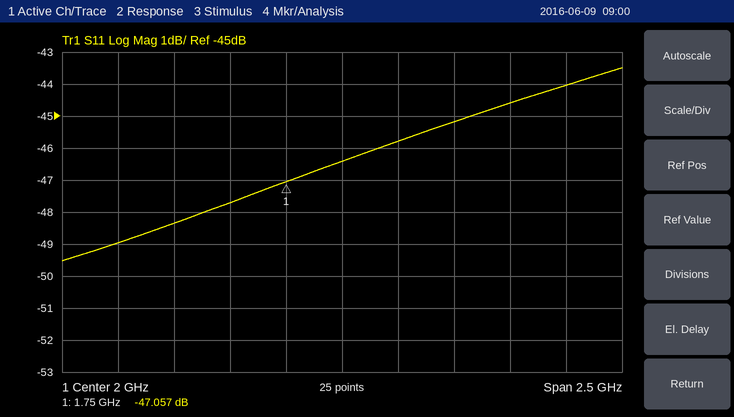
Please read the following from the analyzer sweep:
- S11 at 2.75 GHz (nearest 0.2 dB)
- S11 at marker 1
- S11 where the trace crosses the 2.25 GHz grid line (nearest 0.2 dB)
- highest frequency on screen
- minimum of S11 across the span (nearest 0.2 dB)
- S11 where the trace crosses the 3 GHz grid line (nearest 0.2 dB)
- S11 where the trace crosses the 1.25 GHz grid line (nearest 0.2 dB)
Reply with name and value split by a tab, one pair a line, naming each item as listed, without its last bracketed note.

S11 at 2.75 GHz	-44.6 dB
S11 at marker 1	-47.057 dB
S11 where the trace crosses the 2.25 GHz grid line	-45.8 dB
highest frequency on screen	3.25 GHz
minimum of S11 across the span	-49.6 dB
S11 where the trace crosses the 3 GHz grid line	-44.0 dB
S11 where the trace crosses the 1.25 GHz grid line	-48.4 dB
